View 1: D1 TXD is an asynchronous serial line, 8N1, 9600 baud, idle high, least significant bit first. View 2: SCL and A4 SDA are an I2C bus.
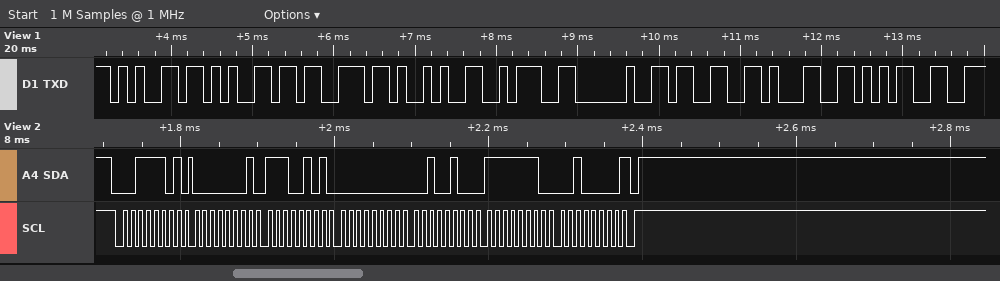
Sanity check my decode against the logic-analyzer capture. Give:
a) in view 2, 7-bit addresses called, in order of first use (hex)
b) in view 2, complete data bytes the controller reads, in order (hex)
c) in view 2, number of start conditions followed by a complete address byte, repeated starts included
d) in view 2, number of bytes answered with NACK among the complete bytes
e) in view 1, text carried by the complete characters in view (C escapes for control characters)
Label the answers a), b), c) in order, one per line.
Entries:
a) 0x1E
b) 01 E5 00 24 FE 20
c) 1
d) 1
e) "ees): 315"
